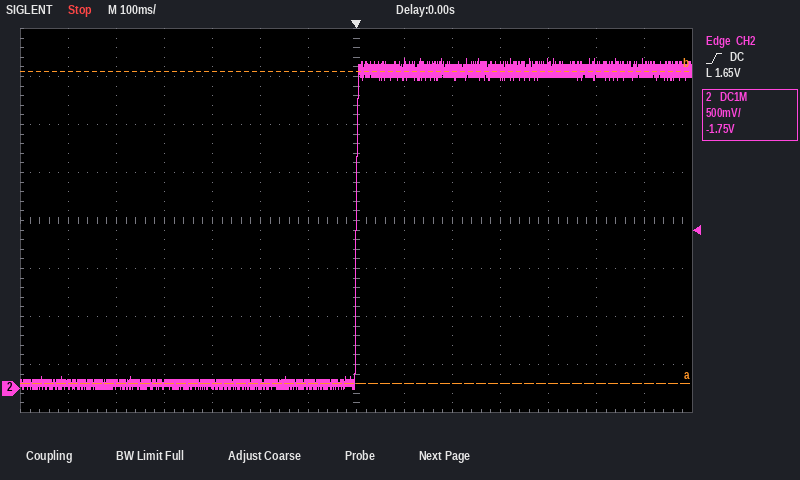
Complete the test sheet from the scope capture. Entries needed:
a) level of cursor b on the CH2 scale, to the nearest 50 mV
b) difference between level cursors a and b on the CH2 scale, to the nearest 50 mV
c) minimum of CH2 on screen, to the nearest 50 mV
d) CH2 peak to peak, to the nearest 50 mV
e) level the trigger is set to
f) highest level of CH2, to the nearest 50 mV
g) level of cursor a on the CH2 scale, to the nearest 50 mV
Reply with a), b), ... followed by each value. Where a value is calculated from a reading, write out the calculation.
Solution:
a) 3.30 V
b) 3.25 V
c) 0 mV
d) 3.45 V − (0 mV) = 3.45 V
e) 1.65 V
f) 3.45 V
g) 50 mV
